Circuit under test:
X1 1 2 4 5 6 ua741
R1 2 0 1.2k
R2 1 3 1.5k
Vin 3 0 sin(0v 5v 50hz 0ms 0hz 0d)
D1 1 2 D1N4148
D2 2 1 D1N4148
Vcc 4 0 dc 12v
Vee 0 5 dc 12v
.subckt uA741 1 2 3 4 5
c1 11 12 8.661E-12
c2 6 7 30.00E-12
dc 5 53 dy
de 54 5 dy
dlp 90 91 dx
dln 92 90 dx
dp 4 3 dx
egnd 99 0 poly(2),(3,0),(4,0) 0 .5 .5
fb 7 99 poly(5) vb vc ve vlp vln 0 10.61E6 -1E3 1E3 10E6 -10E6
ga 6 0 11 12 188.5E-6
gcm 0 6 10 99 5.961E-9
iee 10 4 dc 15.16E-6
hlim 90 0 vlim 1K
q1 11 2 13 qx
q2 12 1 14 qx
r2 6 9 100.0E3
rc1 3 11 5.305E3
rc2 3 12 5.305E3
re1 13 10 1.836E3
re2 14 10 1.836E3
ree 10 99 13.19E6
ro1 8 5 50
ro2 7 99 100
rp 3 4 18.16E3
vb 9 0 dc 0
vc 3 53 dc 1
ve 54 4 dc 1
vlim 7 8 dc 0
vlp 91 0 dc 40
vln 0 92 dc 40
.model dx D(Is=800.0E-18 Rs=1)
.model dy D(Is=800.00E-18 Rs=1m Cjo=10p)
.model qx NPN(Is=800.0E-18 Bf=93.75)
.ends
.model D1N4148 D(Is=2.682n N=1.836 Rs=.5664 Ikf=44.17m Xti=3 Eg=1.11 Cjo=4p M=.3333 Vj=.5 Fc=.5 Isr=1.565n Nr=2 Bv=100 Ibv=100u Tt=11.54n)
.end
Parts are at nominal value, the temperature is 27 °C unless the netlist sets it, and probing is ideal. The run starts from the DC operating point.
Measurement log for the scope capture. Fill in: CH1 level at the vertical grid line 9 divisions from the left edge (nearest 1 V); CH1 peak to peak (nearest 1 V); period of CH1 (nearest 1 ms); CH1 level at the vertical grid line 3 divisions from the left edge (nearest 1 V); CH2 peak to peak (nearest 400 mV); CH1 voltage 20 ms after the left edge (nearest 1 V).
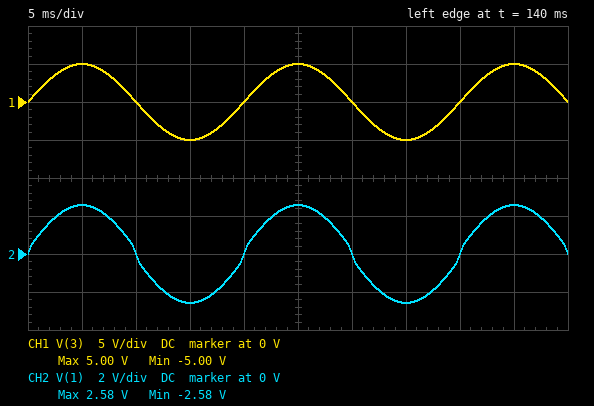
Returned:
5 V
10 V
20 ms
-5 V
5.2 V
0 V
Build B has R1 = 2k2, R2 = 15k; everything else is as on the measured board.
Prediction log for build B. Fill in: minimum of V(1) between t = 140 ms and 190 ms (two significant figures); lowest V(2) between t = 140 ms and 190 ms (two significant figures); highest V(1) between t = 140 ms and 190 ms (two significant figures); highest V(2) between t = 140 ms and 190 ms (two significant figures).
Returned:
-1.1 V
-570 mV
1.1 V
570 mV
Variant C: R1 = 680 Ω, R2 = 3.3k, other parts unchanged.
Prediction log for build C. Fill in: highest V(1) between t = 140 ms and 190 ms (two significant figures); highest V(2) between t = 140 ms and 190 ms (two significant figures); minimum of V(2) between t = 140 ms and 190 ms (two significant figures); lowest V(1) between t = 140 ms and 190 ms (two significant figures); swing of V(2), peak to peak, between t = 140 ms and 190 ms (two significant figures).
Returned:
1.4 V
750 mV
-750 mV
-1.4 V
1.5 V
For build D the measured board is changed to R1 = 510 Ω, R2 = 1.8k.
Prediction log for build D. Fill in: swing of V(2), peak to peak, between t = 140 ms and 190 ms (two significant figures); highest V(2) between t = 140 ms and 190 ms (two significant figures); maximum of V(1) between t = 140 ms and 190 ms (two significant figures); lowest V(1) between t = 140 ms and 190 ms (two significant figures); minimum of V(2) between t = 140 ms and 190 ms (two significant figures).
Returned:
1.9 V
960 mV
1.6 V
-1.6 V
-960 mV
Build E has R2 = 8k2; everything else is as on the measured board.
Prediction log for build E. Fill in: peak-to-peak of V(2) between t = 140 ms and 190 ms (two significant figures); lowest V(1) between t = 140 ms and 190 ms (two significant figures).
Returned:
1.1 V
-1.1 V
